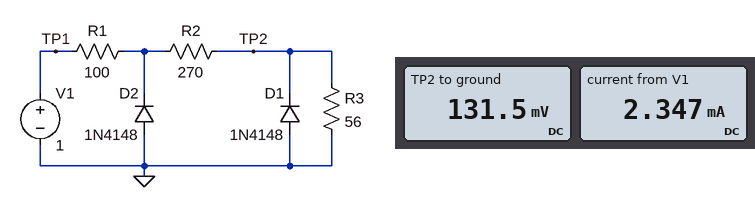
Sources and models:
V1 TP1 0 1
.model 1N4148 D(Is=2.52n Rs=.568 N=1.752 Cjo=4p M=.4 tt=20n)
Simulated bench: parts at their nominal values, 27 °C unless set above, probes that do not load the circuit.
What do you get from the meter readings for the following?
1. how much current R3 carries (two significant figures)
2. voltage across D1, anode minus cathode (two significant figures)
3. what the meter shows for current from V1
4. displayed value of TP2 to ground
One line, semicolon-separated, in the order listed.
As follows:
2.3 mA; -130 mV; 2.347 mA; 131.5 mV
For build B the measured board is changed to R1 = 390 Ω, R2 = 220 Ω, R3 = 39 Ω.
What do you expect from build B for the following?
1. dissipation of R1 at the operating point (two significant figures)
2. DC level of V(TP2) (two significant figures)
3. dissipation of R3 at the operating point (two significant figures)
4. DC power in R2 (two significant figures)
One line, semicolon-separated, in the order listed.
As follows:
930 µW; 60 mV; 93 µW; 520 µW
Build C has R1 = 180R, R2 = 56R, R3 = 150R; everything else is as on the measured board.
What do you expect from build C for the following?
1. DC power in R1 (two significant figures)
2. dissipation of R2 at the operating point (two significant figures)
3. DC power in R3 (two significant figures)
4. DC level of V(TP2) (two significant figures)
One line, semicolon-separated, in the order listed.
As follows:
1.2 mW; 380 µW; 1.0 mW; 390 mV
